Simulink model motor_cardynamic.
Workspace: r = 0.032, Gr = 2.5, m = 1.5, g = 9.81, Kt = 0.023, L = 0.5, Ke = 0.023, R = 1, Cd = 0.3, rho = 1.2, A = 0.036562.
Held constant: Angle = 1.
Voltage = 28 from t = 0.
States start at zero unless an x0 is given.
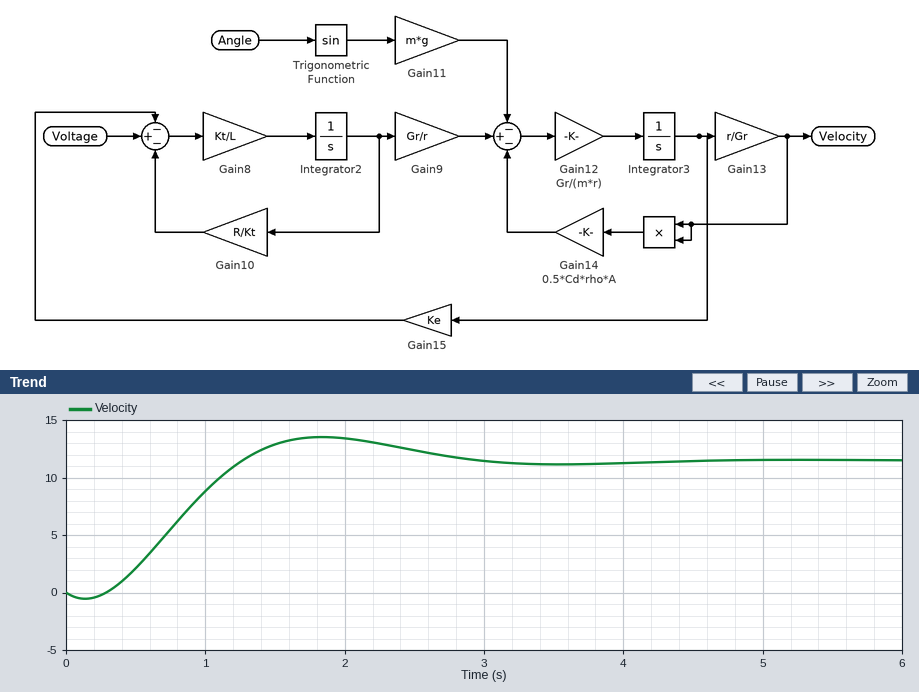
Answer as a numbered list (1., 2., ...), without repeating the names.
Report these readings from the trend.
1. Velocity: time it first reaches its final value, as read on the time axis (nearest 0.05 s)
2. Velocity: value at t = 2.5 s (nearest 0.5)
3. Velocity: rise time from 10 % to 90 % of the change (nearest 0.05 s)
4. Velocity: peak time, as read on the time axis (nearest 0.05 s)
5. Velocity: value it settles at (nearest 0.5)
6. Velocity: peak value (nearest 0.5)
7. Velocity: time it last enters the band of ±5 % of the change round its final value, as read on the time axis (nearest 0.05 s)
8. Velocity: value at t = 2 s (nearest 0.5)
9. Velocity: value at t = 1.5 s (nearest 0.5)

1. 1.25 s
2. 12.5
3. 0.70 s
4. 1.85 s
5. 11.5
6. 13.5
7. 2.65 s
8. 13.5
9. 13.0
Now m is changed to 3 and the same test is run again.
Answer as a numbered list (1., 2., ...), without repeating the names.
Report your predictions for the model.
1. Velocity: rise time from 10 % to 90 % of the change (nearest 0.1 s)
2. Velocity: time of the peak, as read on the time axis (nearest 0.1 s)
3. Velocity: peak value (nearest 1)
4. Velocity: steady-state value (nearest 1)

1. 1.2 s
2. 3.2 s
3. 8
4. 8
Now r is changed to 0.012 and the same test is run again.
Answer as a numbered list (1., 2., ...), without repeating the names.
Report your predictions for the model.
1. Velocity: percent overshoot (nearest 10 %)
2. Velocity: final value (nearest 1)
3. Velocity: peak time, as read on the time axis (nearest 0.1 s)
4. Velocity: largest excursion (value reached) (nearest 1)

1. 60 %
2. 5
3. 0.6 s
4. 8
